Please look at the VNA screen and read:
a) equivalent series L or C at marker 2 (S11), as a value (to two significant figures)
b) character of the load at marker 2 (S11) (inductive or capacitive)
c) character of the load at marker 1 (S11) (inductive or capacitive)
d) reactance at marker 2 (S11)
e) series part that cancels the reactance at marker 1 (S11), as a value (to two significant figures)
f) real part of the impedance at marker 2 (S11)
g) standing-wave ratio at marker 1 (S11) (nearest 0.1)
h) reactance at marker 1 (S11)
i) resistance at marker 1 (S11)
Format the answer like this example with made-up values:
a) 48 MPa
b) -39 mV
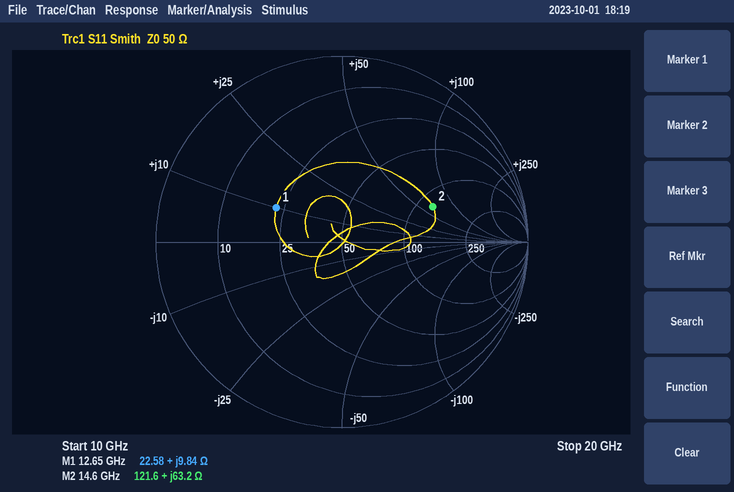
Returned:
a) 690 pH
b) inductive
c) inductive
d) +63.2 Ω
e) 1.3 pF
f) 121.6 Ω
g) 2.3
h) +9.84 Ω
i) 22.58 Ω
